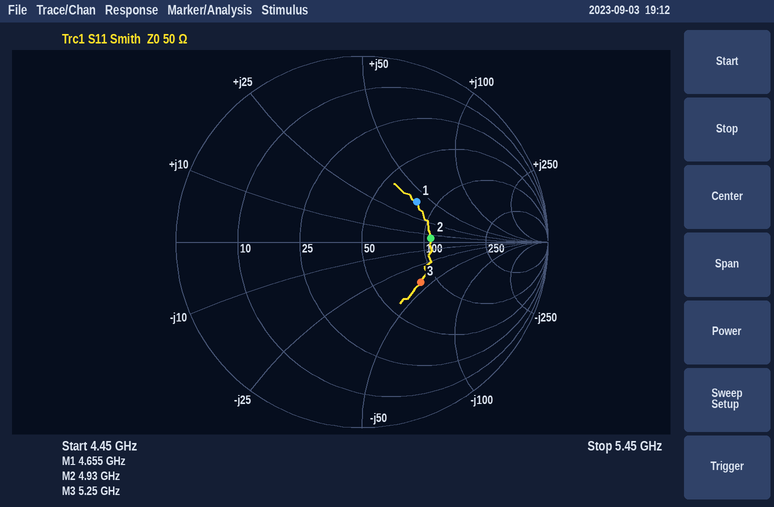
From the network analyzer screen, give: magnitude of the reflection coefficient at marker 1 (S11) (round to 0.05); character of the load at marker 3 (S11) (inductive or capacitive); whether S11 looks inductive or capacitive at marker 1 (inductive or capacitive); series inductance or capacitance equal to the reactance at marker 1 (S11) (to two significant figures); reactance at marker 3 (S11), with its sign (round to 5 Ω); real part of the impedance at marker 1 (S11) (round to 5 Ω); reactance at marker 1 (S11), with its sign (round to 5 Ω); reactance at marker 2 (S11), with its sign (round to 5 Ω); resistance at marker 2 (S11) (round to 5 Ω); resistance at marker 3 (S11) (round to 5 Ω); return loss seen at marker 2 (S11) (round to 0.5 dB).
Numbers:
0.35
capacitive
inductive
1.4 nH
-40 Ω
80 Ω
+40 Ω
+5 Ω
110 Ω
85 Ω
8.5 dB
